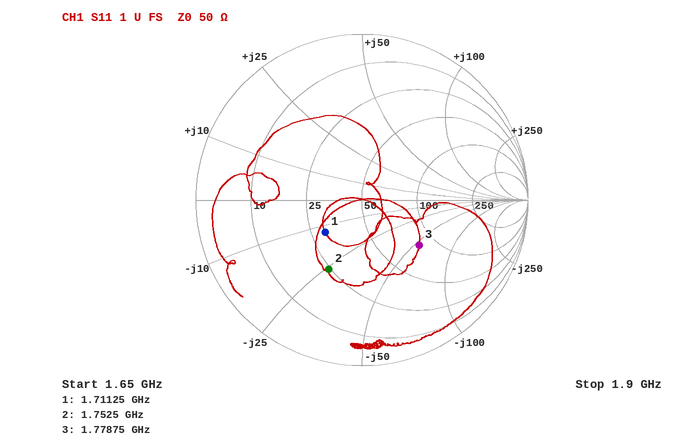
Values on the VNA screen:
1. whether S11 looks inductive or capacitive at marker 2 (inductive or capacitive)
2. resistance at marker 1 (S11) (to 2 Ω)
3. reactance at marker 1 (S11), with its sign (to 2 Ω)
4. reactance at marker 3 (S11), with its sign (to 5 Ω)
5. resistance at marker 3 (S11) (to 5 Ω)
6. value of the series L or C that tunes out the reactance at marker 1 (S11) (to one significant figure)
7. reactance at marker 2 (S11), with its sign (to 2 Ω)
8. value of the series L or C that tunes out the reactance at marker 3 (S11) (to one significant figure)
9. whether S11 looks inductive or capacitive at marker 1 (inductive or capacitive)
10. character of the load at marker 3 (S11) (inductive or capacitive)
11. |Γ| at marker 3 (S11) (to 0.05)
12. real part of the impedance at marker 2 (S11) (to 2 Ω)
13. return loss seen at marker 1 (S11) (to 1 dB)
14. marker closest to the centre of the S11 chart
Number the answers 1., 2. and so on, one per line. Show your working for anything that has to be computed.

1. capacitive
2. 30 Ω
3. -12 Ω
4. -55 Ω
5. 80 Ω
6. L = 12 Ω/(2π × 1.71125 GHz) ≈ 1 nH
7. -26 Ω
8. L = 55 Ω/(2π × 1.77875 GHz) ≈ 5 nH
9. capacitive
10. capacitive
11. 0.45
12. 24 Ω
13. 11 dB
14. marker 1
